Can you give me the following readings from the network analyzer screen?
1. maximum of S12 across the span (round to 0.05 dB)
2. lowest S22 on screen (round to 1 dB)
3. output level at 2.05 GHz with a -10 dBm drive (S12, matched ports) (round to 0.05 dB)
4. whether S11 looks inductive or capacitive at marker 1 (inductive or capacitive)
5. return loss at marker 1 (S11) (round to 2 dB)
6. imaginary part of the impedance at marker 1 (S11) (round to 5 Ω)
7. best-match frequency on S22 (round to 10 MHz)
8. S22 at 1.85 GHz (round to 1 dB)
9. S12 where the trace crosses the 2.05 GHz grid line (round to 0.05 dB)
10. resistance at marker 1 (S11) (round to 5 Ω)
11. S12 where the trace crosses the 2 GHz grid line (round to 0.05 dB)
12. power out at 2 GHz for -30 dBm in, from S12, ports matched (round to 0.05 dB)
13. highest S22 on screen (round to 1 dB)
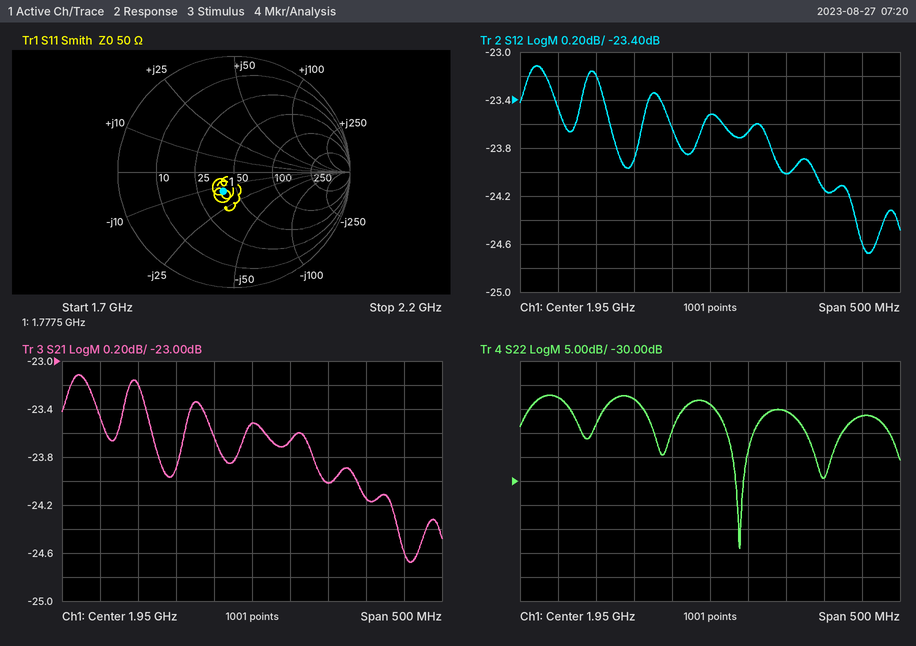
-23.10 dB
-44 dB
-34.00 dBm
capacitive
14 dB
-15 Ω
1.99 GHz
-13 dB
-24.00 dB
40 Ω
-23.65 dB
-53.65 dBm
-12 dB
